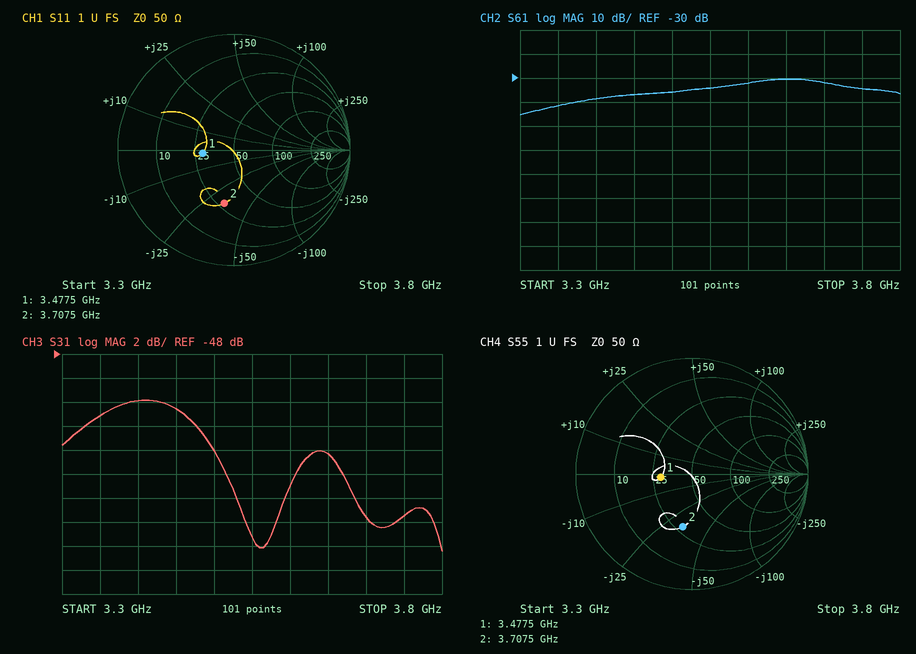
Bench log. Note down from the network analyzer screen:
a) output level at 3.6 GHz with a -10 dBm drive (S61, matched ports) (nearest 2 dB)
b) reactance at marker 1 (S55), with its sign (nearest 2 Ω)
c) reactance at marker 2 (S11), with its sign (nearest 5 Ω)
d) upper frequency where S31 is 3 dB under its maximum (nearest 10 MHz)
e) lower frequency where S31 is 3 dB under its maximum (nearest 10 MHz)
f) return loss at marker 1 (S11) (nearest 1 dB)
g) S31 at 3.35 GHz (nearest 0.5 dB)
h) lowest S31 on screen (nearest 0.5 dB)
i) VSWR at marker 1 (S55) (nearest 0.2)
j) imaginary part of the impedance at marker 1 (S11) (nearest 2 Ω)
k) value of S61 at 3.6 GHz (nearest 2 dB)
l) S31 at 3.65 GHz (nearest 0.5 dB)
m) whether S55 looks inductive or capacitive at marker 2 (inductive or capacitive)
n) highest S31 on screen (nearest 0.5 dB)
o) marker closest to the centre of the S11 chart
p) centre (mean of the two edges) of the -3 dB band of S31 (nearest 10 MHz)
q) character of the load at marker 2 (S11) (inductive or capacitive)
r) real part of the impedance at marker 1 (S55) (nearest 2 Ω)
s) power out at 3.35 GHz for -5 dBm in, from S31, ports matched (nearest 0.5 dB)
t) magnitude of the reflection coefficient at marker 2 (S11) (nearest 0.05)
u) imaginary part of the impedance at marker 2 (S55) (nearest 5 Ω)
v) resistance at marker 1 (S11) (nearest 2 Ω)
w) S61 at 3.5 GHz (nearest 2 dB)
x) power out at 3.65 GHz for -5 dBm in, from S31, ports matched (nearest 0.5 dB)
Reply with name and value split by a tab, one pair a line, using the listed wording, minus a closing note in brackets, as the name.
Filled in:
output level at 3.6 GHz with a -10 dBm drive (S61, matched ports)	-42 dBm
reactance at marker 1 (S55), with its sign	-2 Ω
reactance at marker 2 (S11), with its sign	-35 Ω
upper frequency where S31 is 3 dB under its maximum	3.49 GHz
lower frequency where S31 is 3 dB under its maximum	3.31 GHz
return loss at marker 1 (S11)	11 dB
S31 at 3.35 GHz	-53.0 dB
lowest S31 on screen	-64.5 dB
VSWR at marker 1 (S55)	1.8
imaginary part of the impedance at marker 1 (S11)	-2 Ω
value of S61 at 3.6 GHz	-32 dB
S31 at 3.65 GHz	-56.5 dB
whether S55 looks inductive or capacitive at marker 2	capacitive
highest S31 on screen	-52.0 dB
marker closest to the centre of the S11 chart	marker 1
centre (mean of the two edges) of the -3 dB band of S31	3.40 GHz
character of the load at marker 2 (S11)	capacitive
real part of the impedance at marker 1 (S55)	28 Ω
power out at 3.35 GHz for -5 dBm in, from S31, ports matched	-58.0 dBm
magnitude of the reflection coefficient at marker 2 (S11)	0.45
imaginary part of the impedance at marker 2 (S55)	-35 Ω
resistance at marker 1 (S11)	28 Ω
S61 at 3.5 GHz	-36 dB
power out at 3.65 GHz for -5 dBm in, from S31, ports matched	-61.5 dBm
